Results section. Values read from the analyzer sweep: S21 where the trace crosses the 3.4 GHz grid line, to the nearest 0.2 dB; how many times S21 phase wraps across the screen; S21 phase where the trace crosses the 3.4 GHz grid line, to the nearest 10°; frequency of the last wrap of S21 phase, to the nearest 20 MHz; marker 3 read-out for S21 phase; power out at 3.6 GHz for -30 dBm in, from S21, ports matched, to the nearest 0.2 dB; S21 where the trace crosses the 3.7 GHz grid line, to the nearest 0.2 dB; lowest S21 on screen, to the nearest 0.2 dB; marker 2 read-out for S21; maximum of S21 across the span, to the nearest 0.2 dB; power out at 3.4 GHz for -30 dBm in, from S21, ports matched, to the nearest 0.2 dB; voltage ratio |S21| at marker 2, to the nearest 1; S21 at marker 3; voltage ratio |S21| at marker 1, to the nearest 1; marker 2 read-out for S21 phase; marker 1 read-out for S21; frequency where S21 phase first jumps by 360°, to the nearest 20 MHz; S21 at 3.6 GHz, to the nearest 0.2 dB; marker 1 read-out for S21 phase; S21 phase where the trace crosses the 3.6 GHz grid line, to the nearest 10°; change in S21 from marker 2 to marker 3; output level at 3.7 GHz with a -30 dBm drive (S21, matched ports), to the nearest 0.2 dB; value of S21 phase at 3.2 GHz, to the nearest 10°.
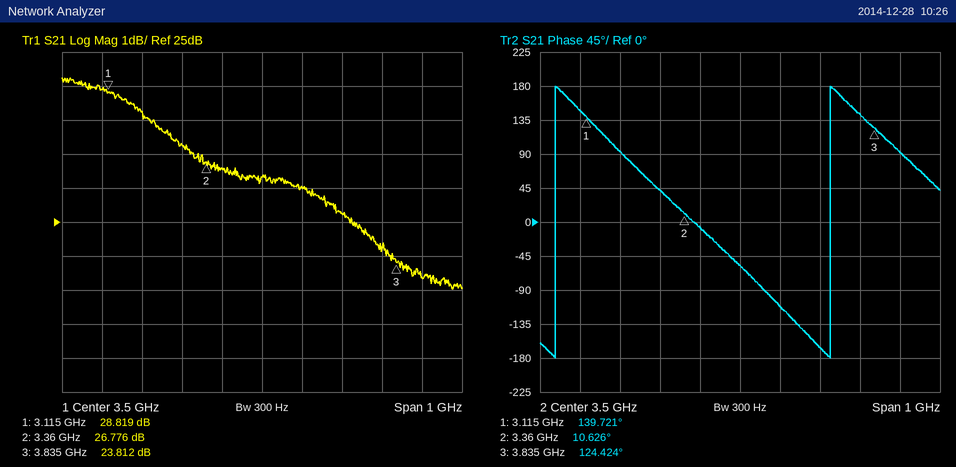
26.6 dB
2
-10°
3.72 GHz
124.424°
-4.0 dBm
25.2 dB
23.0 dB
26.776 dB
29.2 dB
-3.4 dBm
22
23.812 dB
28
10.626°
28.819 dB
3.04 GHz
26.0 dB
139.721°
-110°
-2.964 dB
-4.8 dBm
90°
